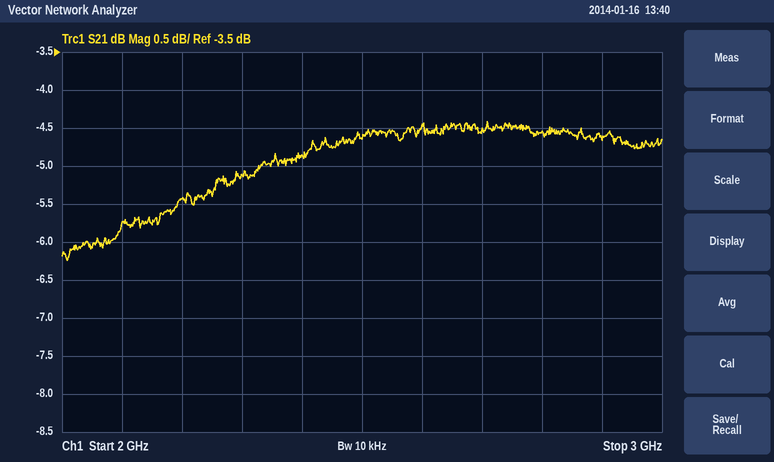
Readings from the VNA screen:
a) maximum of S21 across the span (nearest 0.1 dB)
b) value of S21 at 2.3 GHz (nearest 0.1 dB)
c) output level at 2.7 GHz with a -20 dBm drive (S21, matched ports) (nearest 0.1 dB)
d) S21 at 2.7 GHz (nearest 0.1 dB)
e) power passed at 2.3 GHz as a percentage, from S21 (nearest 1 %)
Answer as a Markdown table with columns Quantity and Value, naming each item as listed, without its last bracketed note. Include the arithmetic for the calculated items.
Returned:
| Quantity | Value |
|---|---|
| maximum of S21 across the span | -4.4 dB |
| value of S21 at 2.3 GHz | -5.1 dB |
| output level at 2.7 GHz with a -20 dBm drive (S21, matched ports) | -20 dBm + (-4.5 dB) = -24.5 dBm |
| S21 at 2.7 GHz | -4.5 dB |
| power passed at 2.3 GHz as a percentage, from S21 | 10^(-5.1/10) ≈ 31 % |
